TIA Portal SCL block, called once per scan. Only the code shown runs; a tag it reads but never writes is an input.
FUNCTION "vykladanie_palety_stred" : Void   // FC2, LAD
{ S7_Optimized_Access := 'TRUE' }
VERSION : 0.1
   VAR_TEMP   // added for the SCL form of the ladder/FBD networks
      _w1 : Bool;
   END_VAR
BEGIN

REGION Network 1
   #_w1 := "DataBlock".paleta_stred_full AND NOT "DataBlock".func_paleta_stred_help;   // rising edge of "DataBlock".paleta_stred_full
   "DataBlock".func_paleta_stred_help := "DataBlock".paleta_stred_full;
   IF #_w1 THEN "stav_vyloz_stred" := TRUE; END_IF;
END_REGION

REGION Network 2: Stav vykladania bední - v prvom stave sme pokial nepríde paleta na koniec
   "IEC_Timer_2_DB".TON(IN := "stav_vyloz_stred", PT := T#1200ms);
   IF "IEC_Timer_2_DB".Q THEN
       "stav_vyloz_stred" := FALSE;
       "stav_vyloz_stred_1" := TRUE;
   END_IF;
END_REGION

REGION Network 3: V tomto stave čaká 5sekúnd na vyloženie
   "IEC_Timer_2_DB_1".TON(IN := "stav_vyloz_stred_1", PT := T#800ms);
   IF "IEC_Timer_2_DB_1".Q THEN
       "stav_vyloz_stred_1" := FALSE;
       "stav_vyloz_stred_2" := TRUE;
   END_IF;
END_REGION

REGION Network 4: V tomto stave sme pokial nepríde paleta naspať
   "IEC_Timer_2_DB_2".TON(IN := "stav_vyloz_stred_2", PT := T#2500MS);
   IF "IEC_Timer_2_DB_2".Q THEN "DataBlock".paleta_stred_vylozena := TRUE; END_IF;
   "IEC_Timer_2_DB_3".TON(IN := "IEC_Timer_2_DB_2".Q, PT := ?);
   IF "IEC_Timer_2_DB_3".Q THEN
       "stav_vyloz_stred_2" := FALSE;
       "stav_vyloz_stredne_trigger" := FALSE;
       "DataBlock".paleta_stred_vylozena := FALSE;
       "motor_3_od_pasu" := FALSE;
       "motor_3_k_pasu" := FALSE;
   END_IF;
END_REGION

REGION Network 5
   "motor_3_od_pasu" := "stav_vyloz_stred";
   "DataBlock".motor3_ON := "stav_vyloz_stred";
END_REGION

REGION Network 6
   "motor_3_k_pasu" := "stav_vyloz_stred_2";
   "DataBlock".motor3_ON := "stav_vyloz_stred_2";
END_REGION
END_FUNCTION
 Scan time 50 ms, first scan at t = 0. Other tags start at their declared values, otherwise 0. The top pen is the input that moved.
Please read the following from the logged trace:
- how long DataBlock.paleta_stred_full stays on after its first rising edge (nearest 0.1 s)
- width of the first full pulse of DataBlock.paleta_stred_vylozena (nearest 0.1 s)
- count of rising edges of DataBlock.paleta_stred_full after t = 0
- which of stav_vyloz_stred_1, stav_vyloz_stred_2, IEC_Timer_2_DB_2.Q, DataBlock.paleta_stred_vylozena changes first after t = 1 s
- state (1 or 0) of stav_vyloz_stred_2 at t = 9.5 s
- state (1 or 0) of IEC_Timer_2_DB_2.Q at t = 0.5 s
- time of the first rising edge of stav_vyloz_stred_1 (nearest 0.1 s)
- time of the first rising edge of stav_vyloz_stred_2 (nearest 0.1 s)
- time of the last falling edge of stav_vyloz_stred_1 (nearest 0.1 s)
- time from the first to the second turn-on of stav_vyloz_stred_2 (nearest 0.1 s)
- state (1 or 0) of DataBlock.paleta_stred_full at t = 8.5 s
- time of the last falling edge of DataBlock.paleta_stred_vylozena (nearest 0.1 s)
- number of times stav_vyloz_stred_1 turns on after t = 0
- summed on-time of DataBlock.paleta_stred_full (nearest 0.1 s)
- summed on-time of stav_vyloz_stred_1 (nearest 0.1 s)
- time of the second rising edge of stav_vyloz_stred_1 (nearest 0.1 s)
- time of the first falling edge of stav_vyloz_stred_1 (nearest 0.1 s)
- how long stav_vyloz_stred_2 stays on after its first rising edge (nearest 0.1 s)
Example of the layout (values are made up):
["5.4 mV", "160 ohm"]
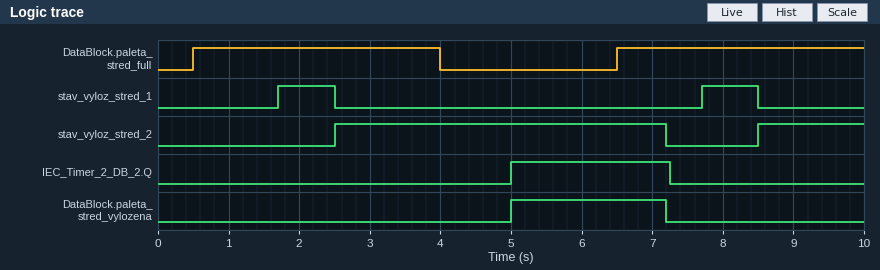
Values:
["3.5 s", "2.2 s", "2", "stav_vyloz_stred_1", "1", "0", "1.7 s", "2.5 s", "8.5 s", "6.0 s", "1", "7.2 s", "2", "7.0 s", "1.6 s", "7.7 s", "2.5 s", "4.7 s"]
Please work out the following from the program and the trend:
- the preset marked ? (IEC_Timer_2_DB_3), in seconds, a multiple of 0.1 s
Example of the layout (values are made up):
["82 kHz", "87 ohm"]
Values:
["2.2 s"]
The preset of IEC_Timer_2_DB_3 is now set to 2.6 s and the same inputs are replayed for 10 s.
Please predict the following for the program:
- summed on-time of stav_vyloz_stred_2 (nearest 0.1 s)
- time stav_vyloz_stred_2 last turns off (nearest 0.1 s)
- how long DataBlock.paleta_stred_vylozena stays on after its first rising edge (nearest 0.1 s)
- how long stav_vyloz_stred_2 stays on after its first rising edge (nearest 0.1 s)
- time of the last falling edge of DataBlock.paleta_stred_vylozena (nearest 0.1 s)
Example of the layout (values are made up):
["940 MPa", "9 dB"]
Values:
["6.6 s", "7.6 s", "2.6 s", "5.1 s", "7.6 s"]
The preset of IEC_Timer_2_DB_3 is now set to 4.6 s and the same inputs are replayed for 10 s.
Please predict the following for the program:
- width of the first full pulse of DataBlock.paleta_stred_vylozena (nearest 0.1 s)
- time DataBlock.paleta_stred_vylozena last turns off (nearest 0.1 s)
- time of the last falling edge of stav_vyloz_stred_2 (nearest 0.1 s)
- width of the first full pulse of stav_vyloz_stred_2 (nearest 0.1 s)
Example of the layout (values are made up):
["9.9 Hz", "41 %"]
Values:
["4.6 s", "9.6 s", "9.6 s", "7.1 s"]
